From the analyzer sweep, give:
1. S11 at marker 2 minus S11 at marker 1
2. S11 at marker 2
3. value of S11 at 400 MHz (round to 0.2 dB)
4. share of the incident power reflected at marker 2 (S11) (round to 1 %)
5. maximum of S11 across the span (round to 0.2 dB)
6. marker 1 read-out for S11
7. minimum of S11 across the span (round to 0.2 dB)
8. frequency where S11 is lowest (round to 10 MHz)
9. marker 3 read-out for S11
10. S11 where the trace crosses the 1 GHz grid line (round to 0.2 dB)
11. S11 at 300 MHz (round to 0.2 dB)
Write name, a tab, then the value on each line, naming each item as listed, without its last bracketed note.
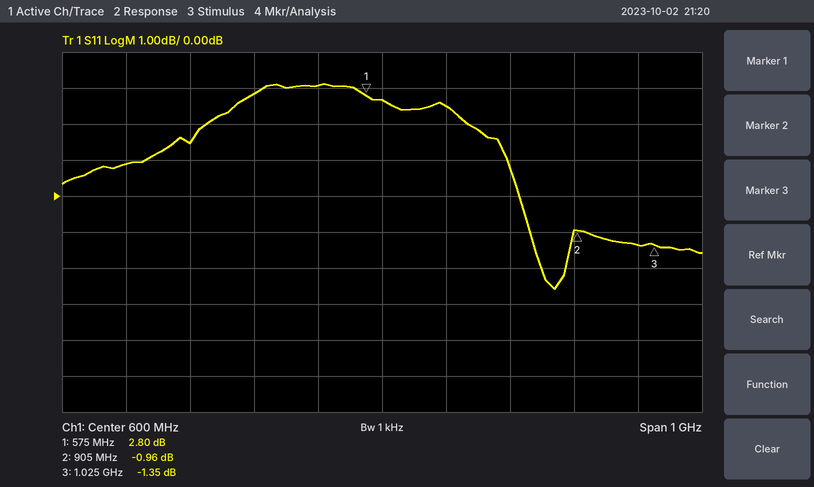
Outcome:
S11 at marker 2 minus S11 at marker 1	-3.76 dB
S11 at marker 2	-0.96 dB
value of S11 at 400 MHz	2.8 dB
share of the incident power reflected at marker 2 (S11)	80 %
maximum of S11 across the span	3.2 dB
marker 1 read-out for S11	2.80 dB
minimum of S11 across the span	-2.6 dB
frequency where S11 is lowest	870 MHz
marker 3 read-out for S11	-1.35 dB
S11 where the trace crosses the 1 GHz grid line	-1.4 dB
S11 at 300 MHz	1.4 dB
